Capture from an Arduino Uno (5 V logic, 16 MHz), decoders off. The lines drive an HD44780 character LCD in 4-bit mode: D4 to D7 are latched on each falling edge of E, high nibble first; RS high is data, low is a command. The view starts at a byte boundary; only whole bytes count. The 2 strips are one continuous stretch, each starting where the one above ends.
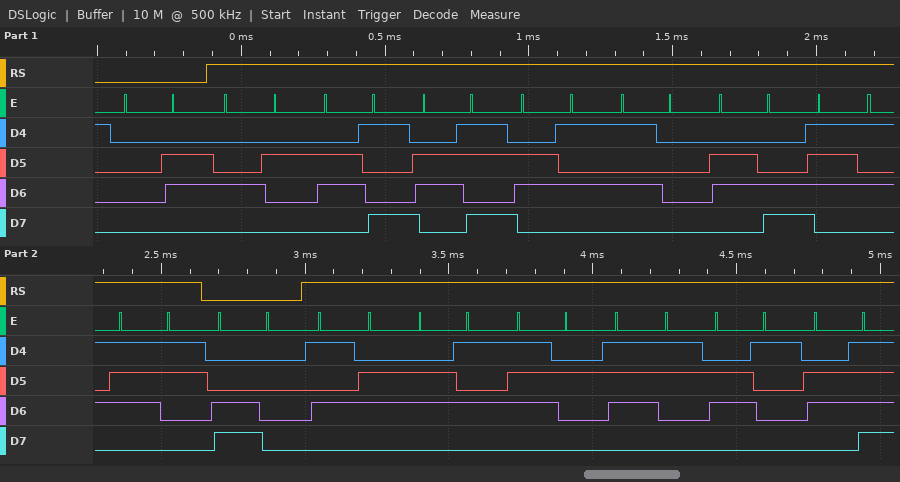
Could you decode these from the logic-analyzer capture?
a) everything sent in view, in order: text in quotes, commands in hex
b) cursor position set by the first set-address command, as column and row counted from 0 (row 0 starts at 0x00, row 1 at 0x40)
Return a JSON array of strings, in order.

["0x06 \"BikePlus\" 0xC0 \"Versao\"", "column 0, row 1"]
